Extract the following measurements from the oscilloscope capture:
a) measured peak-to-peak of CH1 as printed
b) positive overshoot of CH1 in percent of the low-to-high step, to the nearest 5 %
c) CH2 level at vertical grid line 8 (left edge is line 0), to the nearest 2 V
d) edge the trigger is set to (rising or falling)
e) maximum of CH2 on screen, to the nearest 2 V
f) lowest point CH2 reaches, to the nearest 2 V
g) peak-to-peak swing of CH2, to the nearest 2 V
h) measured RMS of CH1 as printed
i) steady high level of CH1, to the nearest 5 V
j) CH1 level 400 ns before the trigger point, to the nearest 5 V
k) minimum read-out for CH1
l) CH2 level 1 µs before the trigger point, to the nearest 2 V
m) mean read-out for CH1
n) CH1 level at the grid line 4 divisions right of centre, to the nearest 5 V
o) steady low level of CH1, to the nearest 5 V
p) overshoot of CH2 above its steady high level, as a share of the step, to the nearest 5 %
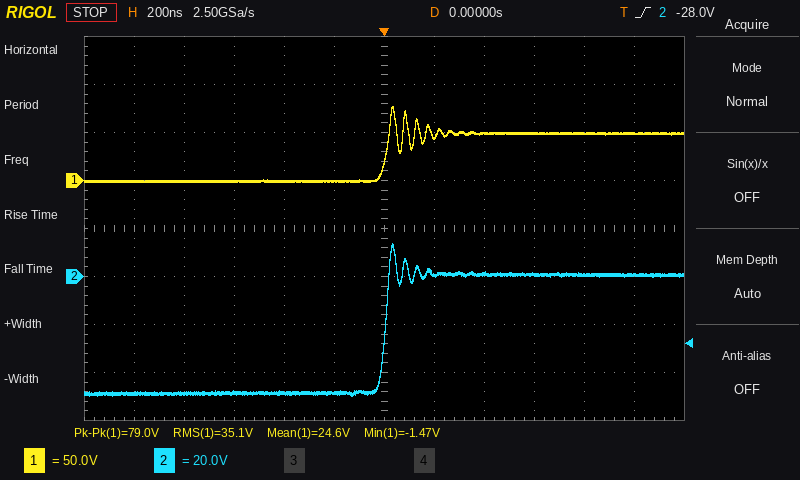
79.0 V
55 %
2 V
rising
14 V
-50 V
64 V
35.1 V
50 V
0 V
-1.47 V
-48 V
24.6 V
50 V
0 V
25 %
